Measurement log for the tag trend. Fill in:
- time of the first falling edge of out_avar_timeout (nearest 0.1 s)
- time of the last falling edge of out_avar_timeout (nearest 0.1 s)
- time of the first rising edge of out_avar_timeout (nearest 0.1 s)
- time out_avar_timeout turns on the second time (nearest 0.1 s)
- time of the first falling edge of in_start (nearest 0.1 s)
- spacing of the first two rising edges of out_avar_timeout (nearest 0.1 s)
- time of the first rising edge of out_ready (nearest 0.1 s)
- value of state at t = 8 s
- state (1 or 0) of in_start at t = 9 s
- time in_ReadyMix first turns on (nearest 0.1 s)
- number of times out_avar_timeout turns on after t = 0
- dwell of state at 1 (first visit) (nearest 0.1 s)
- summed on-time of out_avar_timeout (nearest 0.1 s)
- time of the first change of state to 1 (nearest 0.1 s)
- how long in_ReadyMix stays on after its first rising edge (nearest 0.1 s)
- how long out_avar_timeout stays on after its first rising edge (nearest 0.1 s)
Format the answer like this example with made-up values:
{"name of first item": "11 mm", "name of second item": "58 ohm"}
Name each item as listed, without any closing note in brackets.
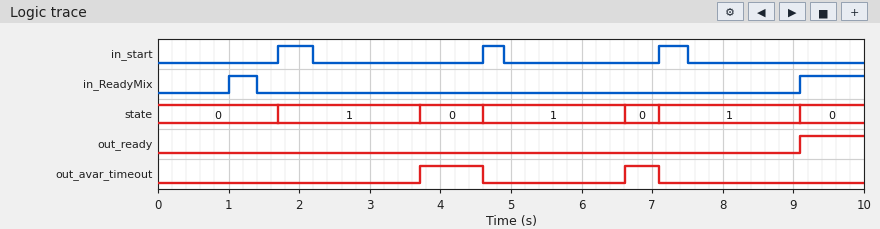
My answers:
{"time of the first falling edge of out_avar_timeout": "4.6 s", "time of the last falling edge of out_avar_timeout": "7.1 s", "time of the first rising edge of out_avar_timeout": "3.7 s", "time out_avar_timeout turns on the second time": "6.6 s", "time of the first falling edge of in_start": "2.2 s", "spacing of the first two rising edges of out_avar_timeout": "2.9 s", "time of the first rising edge of out_ready": "9.1 s", "value of state at t = 8 s": "1", "state (1 or 0) of in_start at t = 9 s": "0", "time in_ReadyMix first turns on": "1.0 s", "number of times out_avar_timeout turns on after t = 0": "2", "dwell of state at 1 (first visit)": "2.0 s", "summed on-time of out_avar_timeout": "1.4 s", "time of the first change of state to 1": "1.7 s", "how long in_ReadyMix stays on after its first rising edge": "0.4 s", "how long out_avar_timeout stays on after its first rising edge": "0.9 s"}
